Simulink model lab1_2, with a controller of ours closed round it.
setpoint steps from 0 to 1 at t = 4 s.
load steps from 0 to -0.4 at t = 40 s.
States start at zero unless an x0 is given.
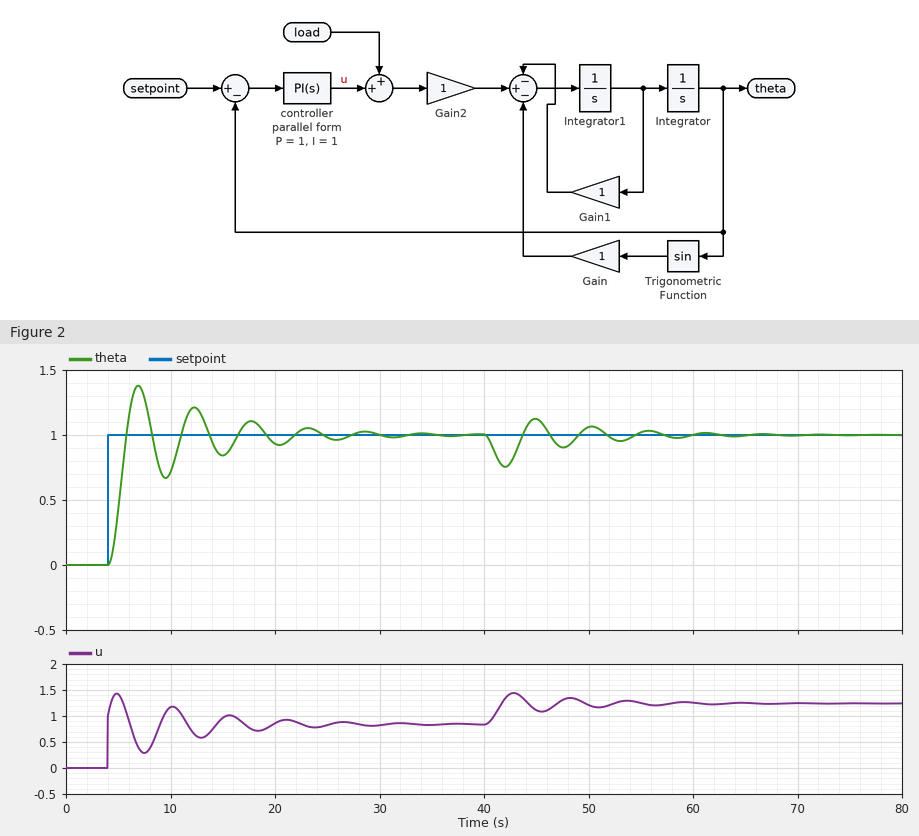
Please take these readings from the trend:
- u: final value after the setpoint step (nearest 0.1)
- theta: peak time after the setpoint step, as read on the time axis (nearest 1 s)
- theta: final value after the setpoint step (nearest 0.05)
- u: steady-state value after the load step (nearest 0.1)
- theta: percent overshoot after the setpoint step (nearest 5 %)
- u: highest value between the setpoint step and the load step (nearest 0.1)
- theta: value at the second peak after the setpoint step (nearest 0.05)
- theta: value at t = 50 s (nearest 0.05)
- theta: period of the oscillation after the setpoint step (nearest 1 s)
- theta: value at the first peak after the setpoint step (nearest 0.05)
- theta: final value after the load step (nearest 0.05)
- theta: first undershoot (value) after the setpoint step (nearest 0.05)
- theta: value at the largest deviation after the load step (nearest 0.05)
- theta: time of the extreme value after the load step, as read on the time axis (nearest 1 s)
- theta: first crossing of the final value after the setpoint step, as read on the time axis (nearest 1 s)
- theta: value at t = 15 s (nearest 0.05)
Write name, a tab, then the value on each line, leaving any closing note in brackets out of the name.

u: final value after the setpoint step	0.8
theta: peak time after the setpoint step, as read on the time axis	7 s
theta: final value after the setpoint step	1.00
u: steady-state value after the load step	1.2
theta: percent overshoot after the setpoint step	40 %
u: highest value between the setpoint step and the load step	1.4
theta: value at the second peak after the setpoint step	1.20
theta: value at t = 50 s	1.05
theta: period of the oscillation after the setpoint step	5 s
theta: value at the first peak after the setpoint step	1.40
theta: final value after the load step	1.00
theta: first undershoot (value) after the setpoint step	0.65
theta: value at the largest deviation after the load step	0.75
theta: time of the extreme value after the load step, as read on the time axis	42 s
theta: first crossing of the final value after the setpoint step, as read on the time axis	6 s
theta: value at t = 15 s	0.85
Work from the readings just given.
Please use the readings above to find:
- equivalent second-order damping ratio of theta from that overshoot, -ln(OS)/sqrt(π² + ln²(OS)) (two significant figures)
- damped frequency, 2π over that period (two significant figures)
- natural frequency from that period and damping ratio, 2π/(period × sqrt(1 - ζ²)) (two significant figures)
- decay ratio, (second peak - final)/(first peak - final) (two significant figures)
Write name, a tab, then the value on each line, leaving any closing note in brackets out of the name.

equivalent second-order damping ratio of theta from that overshoot, -ln(OS)/sqrt(π² + ln²(OS))	0.28
damped frequency, 2π over that period	1.3 rad/s
natural frequency from that period and damping ratio, 2π/(period × sqrt(1 - ζ²))	1.3 rad/s
decay ratio, (second peak - final)/(first peak - final)	0.50
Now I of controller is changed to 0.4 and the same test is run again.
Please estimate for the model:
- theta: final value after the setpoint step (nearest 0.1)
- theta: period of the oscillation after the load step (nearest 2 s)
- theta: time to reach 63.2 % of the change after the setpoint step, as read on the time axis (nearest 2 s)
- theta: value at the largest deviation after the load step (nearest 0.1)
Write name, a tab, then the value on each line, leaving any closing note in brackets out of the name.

theta: final value after the setpoint step	1.0
theta: period of the oscillation after the load step	6 s
theta: time to reach 63.2 % of the change after the setpoint step, as read on the time axis	6 s
theta: value at the largest deviation after the load step	0.7
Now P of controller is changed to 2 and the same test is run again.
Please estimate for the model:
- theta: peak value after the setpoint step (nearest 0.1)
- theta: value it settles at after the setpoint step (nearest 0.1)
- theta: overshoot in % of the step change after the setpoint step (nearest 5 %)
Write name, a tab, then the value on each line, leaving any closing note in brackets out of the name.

theta: peak value after the setpoint step	1.3
theta: value it settles at after the setpoint step	1.0
theta: overshoot in % of the step change after the setpoint step	30 %
